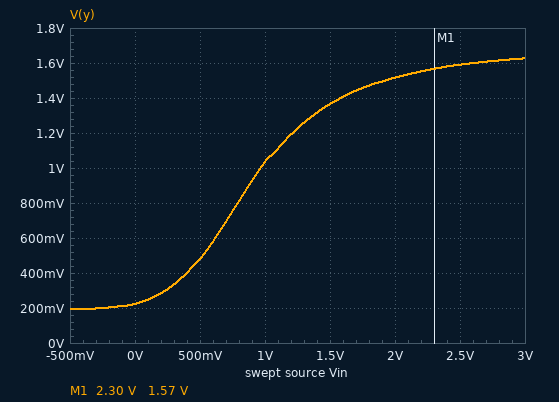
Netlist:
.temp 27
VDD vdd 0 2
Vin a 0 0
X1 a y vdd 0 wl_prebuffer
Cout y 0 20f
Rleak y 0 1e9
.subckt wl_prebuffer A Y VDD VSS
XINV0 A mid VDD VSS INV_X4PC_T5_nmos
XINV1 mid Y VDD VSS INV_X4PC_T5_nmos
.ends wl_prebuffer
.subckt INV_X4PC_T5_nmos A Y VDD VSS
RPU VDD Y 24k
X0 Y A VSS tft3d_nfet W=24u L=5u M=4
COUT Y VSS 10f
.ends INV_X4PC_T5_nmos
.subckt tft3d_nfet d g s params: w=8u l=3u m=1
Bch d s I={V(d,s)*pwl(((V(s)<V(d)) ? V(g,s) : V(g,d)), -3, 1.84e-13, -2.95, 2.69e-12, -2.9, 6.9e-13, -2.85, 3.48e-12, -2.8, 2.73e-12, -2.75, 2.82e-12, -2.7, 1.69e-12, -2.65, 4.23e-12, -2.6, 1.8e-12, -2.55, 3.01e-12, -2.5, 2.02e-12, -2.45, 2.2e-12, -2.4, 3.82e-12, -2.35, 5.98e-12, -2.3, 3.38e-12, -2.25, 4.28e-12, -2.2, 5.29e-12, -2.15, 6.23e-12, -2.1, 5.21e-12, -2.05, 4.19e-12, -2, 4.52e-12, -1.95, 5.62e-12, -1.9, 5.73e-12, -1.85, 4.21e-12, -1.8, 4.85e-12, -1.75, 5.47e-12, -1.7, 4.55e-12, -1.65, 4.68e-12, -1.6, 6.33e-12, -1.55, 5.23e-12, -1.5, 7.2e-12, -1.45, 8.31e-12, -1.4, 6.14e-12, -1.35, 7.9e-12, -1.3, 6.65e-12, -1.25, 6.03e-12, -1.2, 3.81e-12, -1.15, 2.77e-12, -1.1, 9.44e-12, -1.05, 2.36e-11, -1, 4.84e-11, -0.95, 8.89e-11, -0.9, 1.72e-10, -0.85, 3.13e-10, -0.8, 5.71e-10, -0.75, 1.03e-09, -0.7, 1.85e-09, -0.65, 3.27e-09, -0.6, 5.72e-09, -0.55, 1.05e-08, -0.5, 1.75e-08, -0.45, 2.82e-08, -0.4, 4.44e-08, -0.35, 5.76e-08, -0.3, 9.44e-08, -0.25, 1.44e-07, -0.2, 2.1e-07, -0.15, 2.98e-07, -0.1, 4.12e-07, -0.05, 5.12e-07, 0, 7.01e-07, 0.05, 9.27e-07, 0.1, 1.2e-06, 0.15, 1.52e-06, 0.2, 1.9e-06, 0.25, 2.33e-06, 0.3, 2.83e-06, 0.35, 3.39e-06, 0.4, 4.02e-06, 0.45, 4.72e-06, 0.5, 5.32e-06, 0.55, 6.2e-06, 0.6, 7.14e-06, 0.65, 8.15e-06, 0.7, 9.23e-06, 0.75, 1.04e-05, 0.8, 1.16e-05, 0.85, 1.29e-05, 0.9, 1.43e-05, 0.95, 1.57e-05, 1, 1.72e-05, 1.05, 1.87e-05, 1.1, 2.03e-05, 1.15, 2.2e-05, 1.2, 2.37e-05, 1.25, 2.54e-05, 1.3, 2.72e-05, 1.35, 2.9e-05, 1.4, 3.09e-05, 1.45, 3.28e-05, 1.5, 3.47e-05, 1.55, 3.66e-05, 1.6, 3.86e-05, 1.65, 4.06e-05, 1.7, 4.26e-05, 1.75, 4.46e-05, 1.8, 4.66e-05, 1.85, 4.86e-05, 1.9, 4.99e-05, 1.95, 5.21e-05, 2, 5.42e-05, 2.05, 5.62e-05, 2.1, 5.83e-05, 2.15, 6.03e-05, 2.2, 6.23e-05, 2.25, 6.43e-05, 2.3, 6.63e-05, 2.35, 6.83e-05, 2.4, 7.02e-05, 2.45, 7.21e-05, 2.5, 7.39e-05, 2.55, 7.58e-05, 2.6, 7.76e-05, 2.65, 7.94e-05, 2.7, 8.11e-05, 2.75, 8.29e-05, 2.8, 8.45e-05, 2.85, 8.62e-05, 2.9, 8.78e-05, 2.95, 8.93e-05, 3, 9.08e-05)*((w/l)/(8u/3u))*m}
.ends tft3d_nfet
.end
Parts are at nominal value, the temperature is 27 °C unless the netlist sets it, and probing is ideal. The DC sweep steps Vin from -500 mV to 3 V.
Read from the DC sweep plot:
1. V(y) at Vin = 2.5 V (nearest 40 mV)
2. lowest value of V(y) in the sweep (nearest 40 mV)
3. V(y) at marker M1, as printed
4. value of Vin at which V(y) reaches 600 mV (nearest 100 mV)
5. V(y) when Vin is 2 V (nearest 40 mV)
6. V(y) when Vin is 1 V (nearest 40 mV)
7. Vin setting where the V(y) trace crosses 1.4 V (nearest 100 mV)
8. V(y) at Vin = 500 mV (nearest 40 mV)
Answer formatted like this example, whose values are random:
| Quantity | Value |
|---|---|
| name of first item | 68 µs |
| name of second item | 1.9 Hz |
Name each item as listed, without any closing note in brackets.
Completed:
| Quantity | Value |
|---|---|
| V(y) at Vin = 2.5 V | 1.60 V |
| lowest value of V(y) in the sweep | 200 mV |
| V(y) at marker M1, as printed | 1.57 V |
| value of Vin at which V(y) reaches 600 mV | 600 mV |
| V(y) when Vin is 2 V | 1.52 V |
| V(y) when Vin is 1 V | 1.04 V |
| Vin setting where the V(y) trace crosses 1.4 V | 1.6 V |
| V(y) at Vin = 500 mV | 480 mV |
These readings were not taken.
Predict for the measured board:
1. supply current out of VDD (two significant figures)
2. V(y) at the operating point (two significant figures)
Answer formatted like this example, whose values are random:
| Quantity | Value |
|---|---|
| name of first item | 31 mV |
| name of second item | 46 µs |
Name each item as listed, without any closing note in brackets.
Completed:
| Quantity | Value |
|---|---|
| supply current out of VDD | 83 µA |
| V(y) at the operating point | 220 mV |
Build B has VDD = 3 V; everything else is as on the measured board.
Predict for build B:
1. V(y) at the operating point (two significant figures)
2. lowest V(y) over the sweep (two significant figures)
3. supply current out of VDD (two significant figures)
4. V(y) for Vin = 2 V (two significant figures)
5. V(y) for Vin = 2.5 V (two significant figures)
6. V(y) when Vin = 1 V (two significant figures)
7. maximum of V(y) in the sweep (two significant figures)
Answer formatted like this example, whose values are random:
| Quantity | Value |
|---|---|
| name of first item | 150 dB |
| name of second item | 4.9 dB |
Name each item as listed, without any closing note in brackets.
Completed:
| Quantity | Value |
|---|---|
| V(y) at the operating point | 200 mV |
| lowest V(y) over the sweep | 180 mV |
| supply current out of VDD | 130 µA |
| V(y) for Vin = 2 V | 2.0 V |
| V(y) for Vin = 2.5 V | 2.2 V |
| V(y) when Vin = 1 V | 1.1 V |
| maximum of V(y) in the sweep | 2.3 V |
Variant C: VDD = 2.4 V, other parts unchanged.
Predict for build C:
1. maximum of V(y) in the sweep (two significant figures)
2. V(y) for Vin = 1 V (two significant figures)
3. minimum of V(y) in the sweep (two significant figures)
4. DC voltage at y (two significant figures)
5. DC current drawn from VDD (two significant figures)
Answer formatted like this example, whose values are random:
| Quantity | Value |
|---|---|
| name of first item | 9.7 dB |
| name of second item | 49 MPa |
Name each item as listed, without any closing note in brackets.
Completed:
| Quantity | Value |
|---|---|
| maximum of V(y) in the sweep | 1.9 V |
| V(y) for Vin = 1 V | 1.1 V |
| minimum of V(y) in the sweep | 180 mV |
| DC voltage at y | 210 mV |
| DC current drawn from VDD | 100 µA |
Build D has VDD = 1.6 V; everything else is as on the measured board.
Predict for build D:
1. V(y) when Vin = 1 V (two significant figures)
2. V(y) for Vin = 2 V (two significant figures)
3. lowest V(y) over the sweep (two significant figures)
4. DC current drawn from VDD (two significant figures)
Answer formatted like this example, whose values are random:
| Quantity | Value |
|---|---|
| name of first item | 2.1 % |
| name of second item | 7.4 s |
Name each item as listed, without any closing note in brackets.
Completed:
| Quantity | Value |
|---|---|
| V(y) when Vin = 1 V | 940 mV |
| V(y) for Vin = 2 V | 1.3 V |
| lowest V(y) over the sweep | 210 mV |
| DC current drawn from VDD | 64 µA |
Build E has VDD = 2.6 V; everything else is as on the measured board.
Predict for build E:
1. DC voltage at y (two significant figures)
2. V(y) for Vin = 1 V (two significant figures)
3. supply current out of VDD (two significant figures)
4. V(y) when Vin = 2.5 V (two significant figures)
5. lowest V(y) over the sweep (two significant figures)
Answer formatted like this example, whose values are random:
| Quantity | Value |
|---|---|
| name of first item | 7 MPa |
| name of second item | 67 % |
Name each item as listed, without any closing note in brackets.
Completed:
| Quantity | Value |
|---|---|
| DC voltage at y | 210 mV |
| V(y) for Vin = 1 V | 1.1 V |
| supply current out of VDD | 110 µA |
| V(y) when Vin = 2.5 V | 2.0 V |
| lowest V(y) over the sweep | 180 mV |
